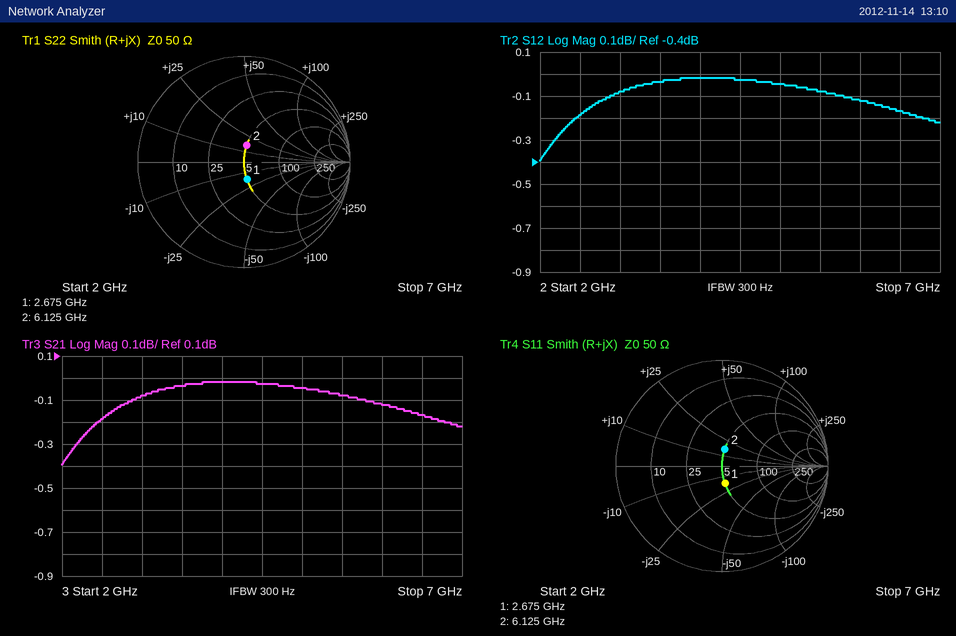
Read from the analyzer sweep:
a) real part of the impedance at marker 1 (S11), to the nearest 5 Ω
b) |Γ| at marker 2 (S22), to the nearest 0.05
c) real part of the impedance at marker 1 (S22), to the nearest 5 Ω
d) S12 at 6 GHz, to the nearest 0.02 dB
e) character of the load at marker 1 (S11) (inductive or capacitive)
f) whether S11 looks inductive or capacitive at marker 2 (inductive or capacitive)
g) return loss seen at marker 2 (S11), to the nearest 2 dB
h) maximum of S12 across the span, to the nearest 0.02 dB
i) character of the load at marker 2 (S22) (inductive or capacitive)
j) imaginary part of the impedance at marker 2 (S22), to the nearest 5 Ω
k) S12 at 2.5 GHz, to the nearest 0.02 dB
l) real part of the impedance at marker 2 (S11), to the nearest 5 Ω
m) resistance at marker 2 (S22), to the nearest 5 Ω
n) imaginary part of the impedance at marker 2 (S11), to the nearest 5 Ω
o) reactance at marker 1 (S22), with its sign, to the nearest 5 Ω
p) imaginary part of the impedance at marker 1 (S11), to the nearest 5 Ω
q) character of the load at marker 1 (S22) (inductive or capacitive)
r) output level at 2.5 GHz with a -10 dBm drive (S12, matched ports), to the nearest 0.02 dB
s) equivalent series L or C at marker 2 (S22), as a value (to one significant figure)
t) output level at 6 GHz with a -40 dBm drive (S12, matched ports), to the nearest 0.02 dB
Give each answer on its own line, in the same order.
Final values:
50 Ω
0.15
50 Ω
-0.12 dB
capacitive
inductive
16 dB
-0.02 dB
inductive
+15 Ω
-0.18 dB
50 Ω
50 Ω
+15 Ω
-15 Ω
-15 Ω
capacitive
-10.18 dBm
400 pH
-40.12 dBm
